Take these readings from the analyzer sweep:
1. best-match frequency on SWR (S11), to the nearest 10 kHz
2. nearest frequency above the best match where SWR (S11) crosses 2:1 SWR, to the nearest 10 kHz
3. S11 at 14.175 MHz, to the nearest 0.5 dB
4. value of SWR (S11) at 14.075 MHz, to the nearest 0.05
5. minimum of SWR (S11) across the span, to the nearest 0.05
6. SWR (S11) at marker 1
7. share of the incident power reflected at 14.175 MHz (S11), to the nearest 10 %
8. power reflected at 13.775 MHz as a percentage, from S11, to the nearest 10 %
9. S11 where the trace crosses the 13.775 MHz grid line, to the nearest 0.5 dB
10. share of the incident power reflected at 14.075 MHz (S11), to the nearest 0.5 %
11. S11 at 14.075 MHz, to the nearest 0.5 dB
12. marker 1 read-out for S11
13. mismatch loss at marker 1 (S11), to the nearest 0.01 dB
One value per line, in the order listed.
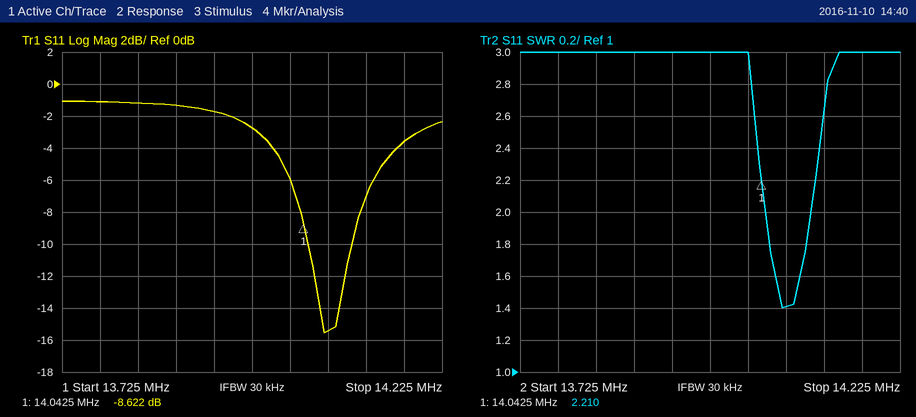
14.07 MHz
14.11 MHz
-3.5 dB
1.40
1.40
2.210
40 %
80 %
-1.0 dB
3.0 %
-15.5 dB
-8.622 dB
0.64 dB
